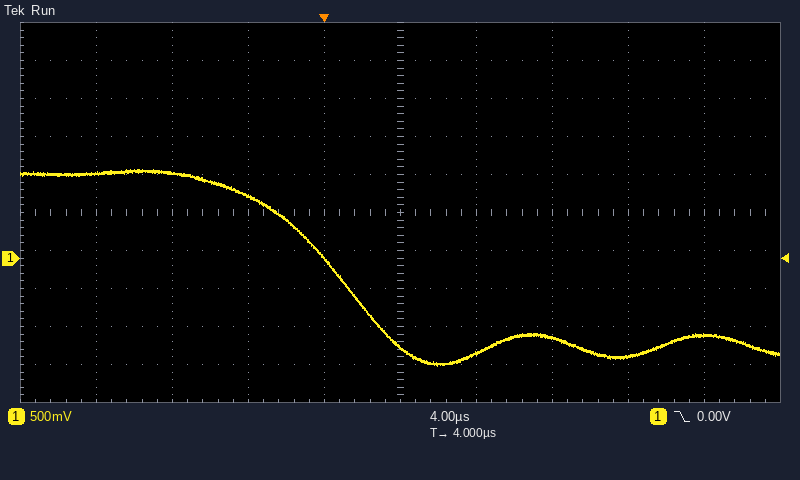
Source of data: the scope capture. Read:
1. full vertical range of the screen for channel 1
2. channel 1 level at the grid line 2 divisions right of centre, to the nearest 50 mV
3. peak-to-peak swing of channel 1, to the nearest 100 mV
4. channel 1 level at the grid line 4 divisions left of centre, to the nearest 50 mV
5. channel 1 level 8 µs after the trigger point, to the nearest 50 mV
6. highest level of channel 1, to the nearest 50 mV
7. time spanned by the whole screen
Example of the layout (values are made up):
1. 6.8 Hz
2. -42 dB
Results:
1. 5 V
2. -1.05 V
3. 2.60 V
4. 1.10 V
5. -1.25 V
6. 1.15 V
7. 40 µs
